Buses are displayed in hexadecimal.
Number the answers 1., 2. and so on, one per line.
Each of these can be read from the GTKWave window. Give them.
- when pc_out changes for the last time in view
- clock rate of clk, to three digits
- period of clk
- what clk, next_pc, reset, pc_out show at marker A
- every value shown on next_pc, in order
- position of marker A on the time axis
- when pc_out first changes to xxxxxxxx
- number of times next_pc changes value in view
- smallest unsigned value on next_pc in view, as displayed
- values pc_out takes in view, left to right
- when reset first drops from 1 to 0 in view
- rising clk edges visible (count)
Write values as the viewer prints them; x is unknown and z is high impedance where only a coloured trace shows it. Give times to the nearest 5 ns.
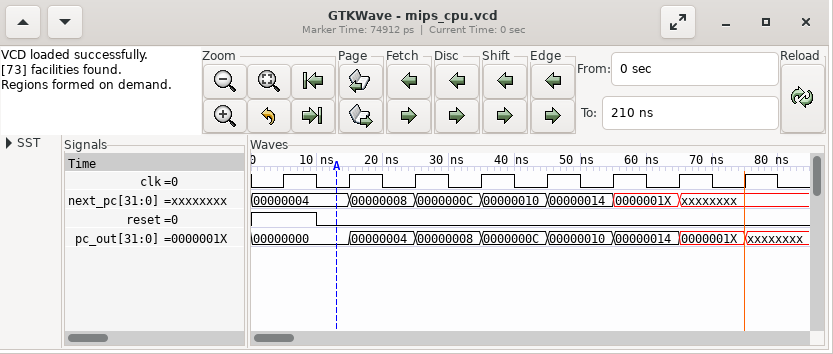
1. 75 ns
2. 100 MHz
3. 10 ns
4. clk=0, next_pc=00000004, reset=0, pc_out=00000000
5. 00000004, 00000008, 0000000C, 00000010, 00000014, 0000001X, xxxxxxxx
6. 15 ns
7. 75 ns
8. 6
9. 00000004
10. 00000000, 00000004, 00000008, 0000000C, 00000010, 00000014, 0000001X, xxxxxxxx
11. 10 ns
12. 8
